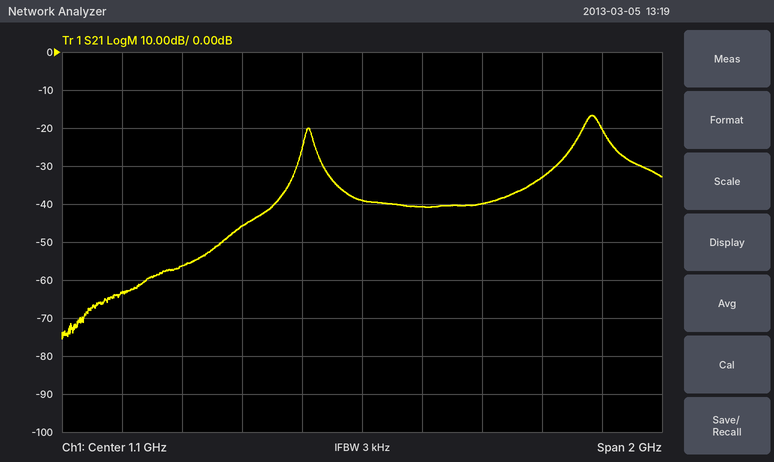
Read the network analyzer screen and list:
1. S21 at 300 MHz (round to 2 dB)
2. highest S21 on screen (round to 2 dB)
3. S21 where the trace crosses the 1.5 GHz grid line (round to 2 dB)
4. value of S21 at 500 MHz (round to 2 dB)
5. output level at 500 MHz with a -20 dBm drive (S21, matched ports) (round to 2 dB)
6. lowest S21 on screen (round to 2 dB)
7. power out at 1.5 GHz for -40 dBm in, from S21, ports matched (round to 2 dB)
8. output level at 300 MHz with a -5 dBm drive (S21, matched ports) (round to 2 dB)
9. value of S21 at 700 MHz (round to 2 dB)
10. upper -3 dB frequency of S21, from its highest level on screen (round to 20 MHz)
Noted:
-64 dB
-16 dB
-40 dB
-56 dB
-76 dBm
-76 dB
-80 dBm
-68 dBm
-46 dB
1.90 GHz
